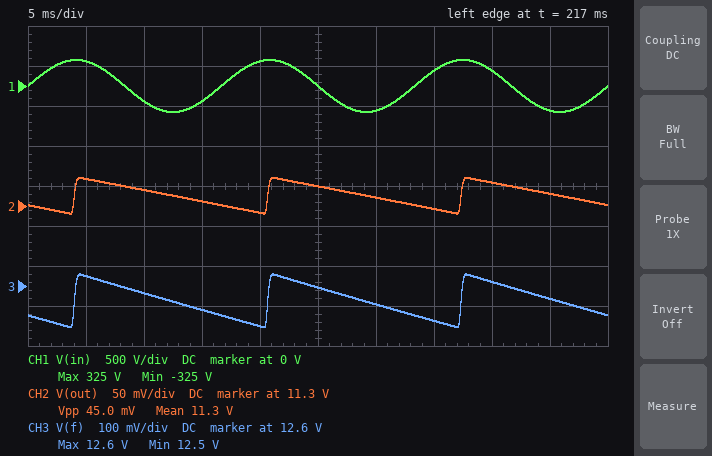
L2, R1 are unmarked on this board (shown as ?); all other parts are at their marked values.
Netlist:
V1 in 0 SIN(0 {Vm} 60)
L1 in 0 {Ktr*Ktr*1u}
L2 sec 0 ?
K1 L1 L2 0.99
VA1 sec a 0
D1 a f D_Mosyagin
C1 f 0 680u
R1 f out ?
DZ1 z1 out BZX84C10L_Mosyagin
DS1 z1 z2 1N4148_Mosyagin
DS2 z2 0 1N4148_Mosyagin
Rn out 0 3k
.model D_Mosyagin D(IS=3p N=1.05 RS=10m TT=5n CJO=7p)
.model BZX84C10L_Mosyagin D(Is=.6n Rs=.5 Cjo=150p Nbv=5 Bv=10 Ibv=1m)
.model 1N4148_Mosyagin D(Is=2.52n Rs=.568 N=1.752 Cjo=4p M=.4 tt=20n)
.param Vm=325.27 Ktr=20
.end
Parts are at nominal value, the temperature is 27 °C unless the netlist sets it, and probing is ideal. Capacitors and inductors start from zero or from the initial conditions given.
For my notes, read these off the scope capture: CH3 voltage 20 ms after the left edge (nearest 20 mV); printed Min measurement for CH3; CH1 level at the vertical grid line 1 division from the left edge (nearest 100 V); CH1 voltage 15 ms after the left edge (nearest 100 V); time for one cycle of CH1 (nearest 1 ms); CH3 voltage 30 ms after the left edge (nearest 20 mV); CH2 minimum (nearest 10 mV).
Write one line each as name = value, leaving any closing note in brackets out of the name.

CH3 voltage 20 ms after the left edge = 12.50 V
printed Min measurement for CH3 = 12.5 V
CH1 level at the vertical grid line 1 division from the left edge = 300 V
CH1 voltage 15 ms after the left edge = -200 V
time for one cycle of CH1 = 17 ms
CH3 voltage 30 ms after the left edge = 12.56 V
CH2 minimum = 11.29 V
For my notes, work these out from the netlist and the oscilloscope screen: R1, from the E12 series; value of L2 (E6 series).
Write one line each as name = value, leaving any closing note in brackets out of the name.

R1, from the E12 series = 220 Ω
value of L2 = 680 nH
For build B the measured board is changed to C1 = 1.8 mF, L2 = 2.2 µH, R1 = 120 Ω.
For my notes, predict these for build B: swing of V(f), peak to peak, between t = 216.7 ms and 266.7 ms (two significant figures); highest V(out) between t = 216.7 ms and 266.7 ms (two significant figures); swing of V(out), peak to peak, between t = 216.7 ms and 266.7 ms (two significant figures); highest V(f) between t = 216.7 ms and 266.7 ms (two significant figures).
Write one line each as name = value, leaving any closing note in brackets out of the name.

swing of V(f), peak to peak, between t = 216.7 ms and 266.7 ms = 770 mV
highest V(out) between t = 216.7 ms and 266.7 ms = 12 V
swing of V(out), peak to peak, between t = 216.7 ms and 266.7 ms = 26 mV
highest V(f) between t = 216.7 ms and 266.7 ms = 23 V
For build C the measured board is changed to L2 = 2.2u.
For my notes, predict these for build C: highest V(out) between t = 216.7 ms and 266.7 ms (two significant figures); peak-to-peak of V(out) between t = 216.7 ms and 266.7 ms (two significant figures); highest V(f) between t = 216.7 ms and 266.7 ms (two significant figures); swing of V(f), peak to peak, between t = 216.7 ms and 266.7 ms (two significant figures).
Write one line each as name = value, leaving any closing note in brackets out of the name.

highest V(out) between t = 216.7 ms and 266.7 ms = 12 V
peak-to-peak of V(out) between t = 216.7 ms and 266.7 ms = 32 mV
highest V(f) between t = 216.7 ms and 266.7 ms = 23 V
swing of V(f), peak to peak, between t = 216.7 ms and 266.7 ms = 1.1 V
